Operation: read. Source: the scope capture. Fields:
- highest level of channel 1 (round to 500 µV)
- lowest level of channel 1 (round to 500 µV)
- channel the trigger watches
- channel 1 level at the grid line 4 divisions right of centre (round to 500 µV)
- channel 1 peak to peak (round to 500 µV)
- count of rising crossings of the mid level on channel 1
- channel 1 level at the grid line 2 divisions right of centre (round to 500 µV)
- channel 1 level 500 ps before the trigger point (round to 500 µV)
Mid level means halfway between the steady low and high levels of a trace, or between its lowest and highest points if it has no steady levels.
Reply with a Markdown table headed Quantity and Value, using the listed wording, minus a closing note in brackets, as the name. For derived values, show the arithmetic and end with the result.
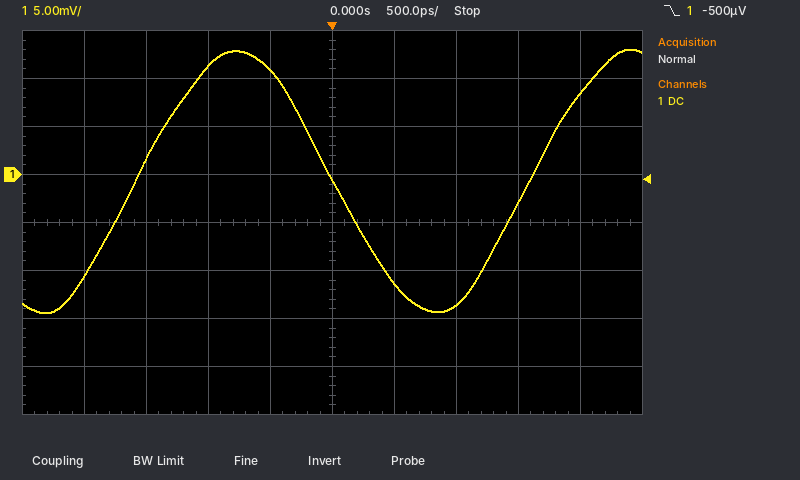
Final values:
| Quantity | Value |
|---|---|
| highest level of channel 1 | 13.0 mV |
| lowest level of channel 1 | -14.5 mV |
| channel the trigger watches | channel 1 |
| channel 1 level at the grid line 4 divisions right of centre | 8.5 mV |
| channel 1 peak to peak | 13.0 mV − (-14.5 mV) = 27.5 mV |
| count of rising crossings of the mid level on channel 1 | 2 |
| channel 1 level at the grid line 2 divisions right of centre | -13.5 mV |
| channel 1 level 500 ps before the trigger point | 11.0 mV |
